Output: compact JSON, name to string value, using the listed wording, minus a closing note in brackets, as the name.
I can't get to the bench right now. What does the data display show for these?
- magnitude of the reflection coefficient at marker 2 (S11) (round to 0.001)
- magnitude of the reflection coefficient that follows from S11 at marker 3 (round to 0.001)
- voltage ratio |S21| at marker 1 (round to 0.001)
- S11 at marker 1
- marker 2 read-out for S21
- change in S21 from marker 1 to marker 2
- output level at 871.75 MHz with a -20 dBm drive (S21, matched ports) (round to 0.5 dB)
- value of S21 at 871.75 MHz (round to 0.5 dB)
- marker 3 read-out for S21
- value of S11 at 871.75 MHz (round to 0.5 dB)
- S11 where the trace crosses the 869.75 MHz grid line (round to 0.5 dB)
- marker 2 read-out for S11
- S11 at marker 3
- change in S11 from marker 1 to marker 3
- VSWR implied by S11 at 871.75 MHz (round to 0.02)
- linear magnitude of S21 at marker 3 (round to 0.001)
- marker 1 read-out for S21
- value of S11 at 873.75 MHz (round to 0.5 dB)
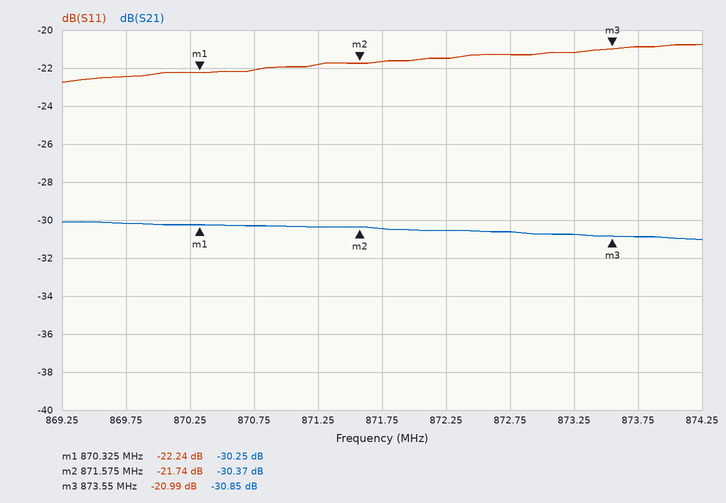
{"magnitude of the reflection coefficient at marker 2 (S11)": "0.082", "magnitude of the reflection coefficient that follows from S11 at marker 3": "0.089", "voltage ratio |S21| at marker 1": "0.031", "S11 at marker 1": "-22.24 dB", "marker 2 read-out for S21": "-30.37 dB", "change in S21 from marker 1 to marker 2": "-0.12 dB", "output level at 871.75 MHz with a -20 dBm drive (S21, matched ports)": "-50.5 dBm", "value of S21 at 871.75 MHz": "-30.5 dB", "marker 3 read-out for S21": "-30.85 dB", "value of S11 at 871.75 MHz": "-21.5 dB", "S11 where the trace crosses the 869.75 MHz grid line": "-22.5 dB", "marker 2 read-out for S11": "-21.74 dB", "S11 at marker 3": "-20.99 dB", "change in S11 from marker 1 to marker 3": "1.25 dB", "VSWR implied by S11 at 871.75 MHz": "1.18", "linear magnitude of S21 at marker 3": "0.029", "marker 1 read-out for S21": "-30.25 dB", "value of S11 at 873.75 MHz": "-21.0 dB"}
